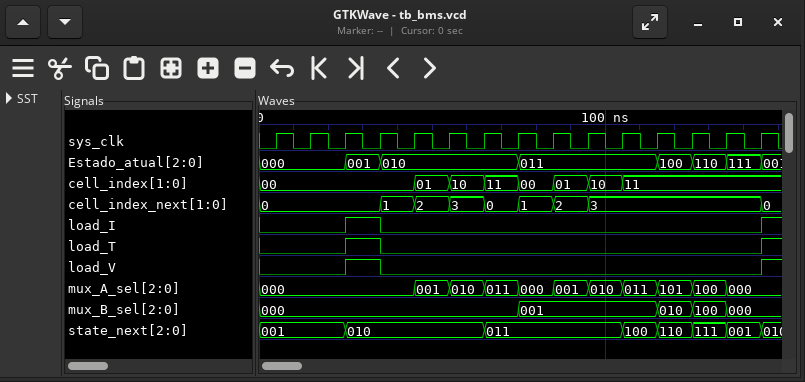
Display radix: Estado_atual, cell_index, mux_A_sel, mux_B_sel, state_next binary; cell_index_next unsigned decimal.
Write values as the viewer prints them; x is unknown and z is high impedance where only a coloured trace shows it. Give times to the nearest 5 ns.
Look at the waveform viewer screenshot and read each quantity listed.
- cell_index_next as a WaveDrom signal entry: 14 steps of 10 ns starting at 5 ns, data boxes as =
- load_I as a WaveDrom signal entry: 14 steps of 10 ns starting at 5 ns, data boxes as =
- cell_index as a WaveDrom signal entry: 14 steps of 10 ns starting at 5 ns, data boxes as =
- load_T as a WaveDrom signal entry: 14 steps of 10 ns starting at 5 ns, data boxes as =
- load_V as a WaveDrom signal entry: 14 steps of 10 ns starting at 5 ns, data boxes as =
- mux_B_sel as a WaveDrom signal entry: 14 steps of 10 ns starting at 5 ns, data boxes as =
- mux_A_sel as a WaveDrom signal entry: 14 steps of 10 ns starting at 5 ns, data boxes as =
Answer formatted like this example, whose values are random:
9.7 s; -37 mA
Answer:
{name: 'cell_index_next', wave: '=..=======....', data: '0 1 2 3 0 1 2 3'}; {name: 'load_I', wave: '0.10..........'}; {name: 'cell_index', wave: '=...=======...', data: '00 01 10 11 00 01 10 11'}; {name: 'load_T', wave: '0.10..........'}; {name: 'load_V', wave: '0.10..........'}; {name: 'mux_B_sel', wave: '=......=...===', data: '000 001 010 100 000'}; {name: 'mux_A_sel', wave: '=...==========', data: '000 001 010 011 000 001 010 011 101 100 000'}
